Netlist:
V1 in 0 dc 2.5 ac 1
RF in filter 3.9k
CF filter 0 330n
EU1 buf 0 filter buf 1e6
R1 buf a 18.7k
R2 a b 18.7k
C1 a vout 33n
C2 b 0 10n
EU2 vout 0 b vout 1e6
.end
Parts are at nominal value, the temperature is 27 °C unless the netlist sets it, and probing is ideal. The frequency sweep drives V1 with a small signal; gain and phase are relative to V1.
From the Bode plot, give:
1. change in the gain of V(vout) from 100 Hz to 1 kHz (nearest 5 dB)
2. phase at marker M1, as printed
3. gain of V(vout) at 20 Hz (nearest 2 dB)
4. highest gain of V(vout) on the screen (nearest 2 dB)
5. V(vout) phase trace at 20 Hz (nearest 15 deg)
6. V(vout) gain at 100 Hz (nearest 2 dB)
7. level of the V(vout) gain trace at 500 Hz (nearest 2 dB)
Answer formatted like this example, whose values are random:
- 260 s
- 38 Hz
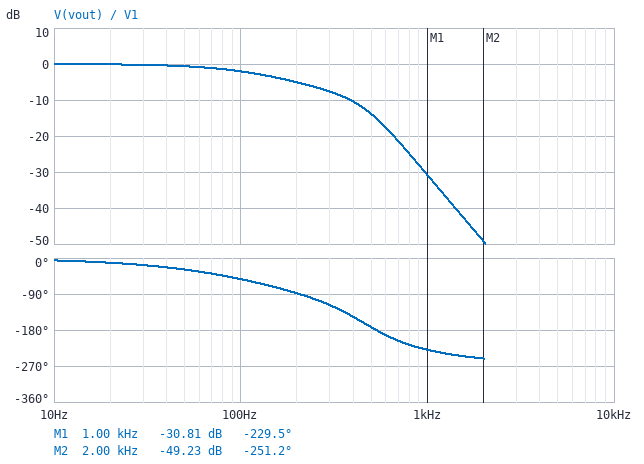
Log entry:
- -30 dB
- -229.5 deg
- 0 dB
- 0 dB
- -15 deg
- -2 dB
- -14 dB
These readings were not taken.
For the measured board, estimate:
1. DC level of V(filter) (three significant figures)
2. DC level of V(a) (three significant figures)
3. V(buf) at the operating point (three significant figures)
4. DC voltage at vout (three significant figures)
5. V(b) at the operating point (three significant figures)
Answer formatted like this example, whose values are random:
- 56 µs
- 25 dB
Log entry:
- 2.50 V
- 2.50 V
- 2.50 V
- 2.50 V
- 2.50 V
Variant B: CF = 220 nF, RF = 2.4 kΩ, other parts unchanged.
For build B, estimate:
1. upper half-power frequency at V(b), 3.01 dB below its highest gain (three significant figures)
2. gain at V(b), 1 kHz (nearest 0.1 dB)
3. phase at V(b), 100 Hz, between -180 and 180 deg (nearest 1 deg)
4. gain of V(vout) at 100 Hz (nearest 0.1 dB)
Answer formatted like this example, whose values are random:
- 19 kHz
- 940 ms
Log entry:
- 345 Hz
- -23.4 dB
- -32 deg
- -0.3 dB
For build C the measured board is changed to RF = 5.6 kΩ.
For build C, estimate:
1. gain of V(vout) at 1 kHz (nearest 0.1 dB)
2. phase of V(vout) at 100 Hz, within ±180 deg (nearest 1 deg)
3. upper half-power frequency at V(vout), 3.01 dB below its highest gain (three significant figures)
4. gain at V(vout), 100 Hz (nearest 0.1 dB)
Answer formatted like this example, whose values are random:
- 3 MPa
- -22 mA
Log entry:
- -33.9 dB
- -63 deg
- 88.5 Hz
- -3.6 dB
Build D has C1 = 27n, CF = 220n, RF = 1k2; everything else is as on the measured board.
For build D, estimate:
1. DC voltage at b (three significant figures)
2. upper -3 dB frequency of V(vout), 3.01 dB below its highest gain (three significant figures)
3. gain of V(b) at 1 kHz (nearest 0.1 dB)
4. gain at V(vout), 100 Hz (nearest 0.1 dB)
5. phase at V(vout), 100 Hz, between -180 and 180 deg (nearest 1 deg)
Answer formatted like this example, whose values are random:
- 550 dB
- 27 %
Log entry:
- 2.50 V
- 469 Hz
- -16.9 dB
- 0 dB
- -23 deg
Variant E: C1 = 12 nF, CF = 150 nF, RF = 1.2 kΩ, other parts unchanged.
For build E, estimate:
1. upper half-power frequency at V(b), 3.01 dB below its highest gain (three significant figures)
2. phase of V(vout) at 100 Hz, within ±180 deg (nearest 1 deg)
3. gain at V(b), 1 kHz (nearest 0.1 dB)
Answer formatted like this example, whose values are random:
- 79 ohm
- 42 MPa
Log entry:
- 456 Hz
- -20 deg
- -11.3 dB
